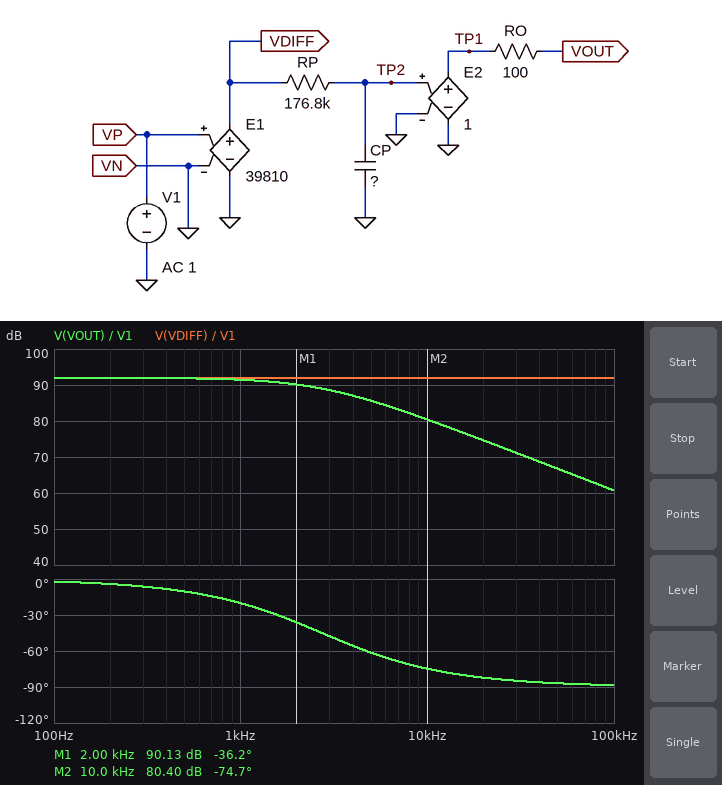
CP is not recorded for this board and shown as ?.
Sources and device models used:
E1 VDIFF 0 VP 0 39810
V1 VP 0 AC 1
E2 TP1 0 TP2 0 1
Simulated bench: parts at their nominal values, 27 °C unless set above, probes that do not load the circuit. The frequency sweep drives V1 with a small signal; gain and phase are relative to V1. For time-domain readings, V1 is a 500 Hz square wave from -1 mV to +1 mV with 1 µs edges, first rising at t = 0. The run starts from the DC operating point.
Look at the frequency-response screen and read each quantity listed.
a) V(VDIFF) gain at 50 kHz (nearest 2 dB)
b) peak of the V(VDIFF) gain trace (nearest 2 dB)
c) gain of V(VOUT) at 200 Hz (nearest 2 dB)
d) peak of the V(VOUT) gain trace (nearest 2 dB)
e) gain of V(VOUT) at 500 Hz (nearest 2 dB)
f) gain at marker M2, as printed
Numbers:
92 dB
92 dB
92 dB
92 dB
92 dB
80.40 dB
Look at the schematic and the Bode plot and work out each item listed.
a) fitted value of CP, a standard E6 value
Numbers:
330 pF
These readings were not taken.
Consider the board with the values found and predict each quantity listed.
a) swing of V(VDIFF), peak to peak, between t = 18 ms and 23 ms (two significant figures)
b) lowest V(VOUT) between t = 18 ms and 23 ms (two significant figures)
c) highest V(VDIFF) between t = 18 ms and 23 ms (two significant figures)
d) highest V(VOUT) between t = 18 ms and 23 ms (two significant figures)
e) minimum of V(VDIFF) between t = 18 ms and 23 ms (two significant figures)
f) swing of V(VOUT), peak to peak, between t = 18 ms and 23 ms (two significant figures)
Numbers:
80 V
-40 V
40 V
40 V
-40 V
80 V
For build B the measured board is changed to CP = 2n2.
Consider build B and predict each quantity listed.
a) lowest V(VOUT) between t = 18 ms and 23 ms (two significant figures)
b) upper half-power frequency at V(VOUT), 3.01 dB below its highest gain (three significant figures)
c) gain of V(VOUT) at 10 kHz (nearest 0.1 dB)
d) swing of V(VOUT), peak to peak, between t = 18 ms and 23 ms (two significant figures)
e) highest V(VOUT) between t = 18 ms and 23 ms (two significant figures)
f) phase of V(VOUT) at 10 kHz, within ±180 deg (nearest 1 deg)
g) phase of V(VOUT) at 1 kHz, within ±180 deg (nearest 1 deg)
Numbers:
-34 V
409 Hz
64.2 dB
68 V
34 V
-88 deg
-68 deg
